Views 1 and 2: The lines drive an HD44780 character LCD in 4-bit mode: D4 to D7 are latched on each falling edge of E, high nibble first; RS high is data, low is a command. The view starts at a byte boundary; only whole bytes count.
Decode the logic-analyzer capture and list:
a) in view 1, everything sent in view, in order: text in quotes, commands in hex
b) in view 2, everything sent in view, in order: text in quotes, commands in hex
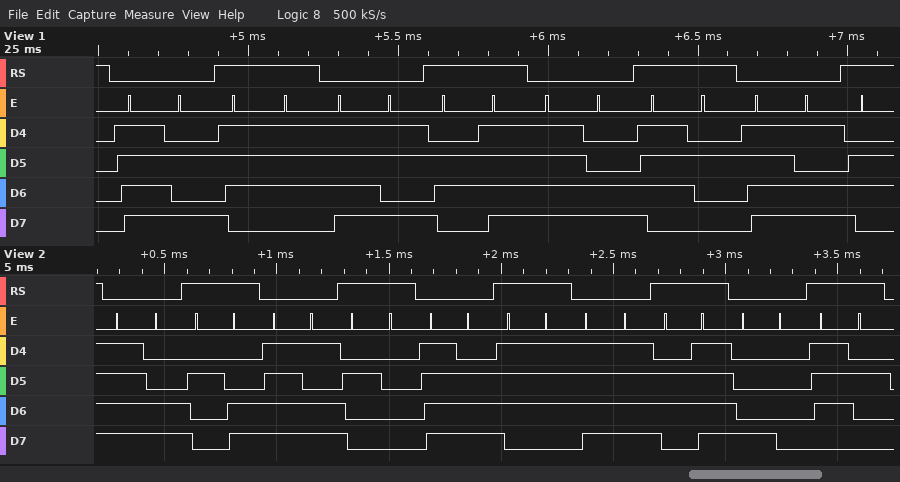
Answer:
0xFA "w" 0xFB "o" 0xFC "r" 0xFD
0xFC "," 0xFD " " 0xFE "w" 0xFF "o" 0x80 "r"
